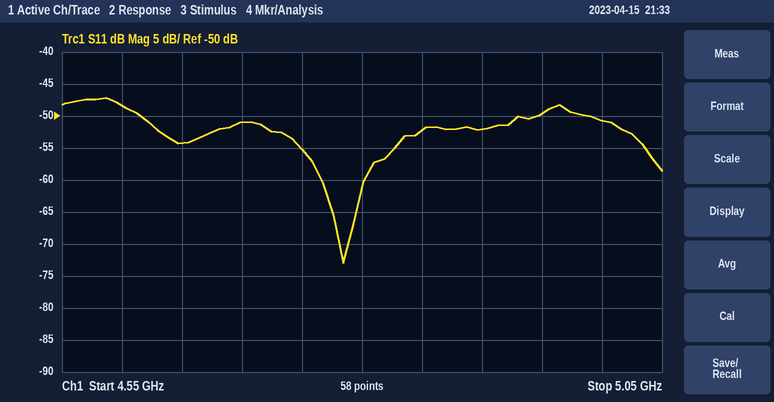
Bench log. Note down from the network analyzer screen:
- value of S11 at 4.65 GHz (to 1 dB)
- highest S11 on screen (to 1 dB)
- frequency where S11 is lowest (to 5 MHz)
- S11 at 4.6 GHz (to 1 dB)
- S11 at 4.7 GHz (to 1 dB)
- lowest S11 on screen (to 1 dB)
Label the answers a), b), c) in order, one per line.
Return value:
a) -54 dB
b) -47 dB
c) 4.785 GHz
d) -48 dB
e) -51 dB
f) -73 dB
